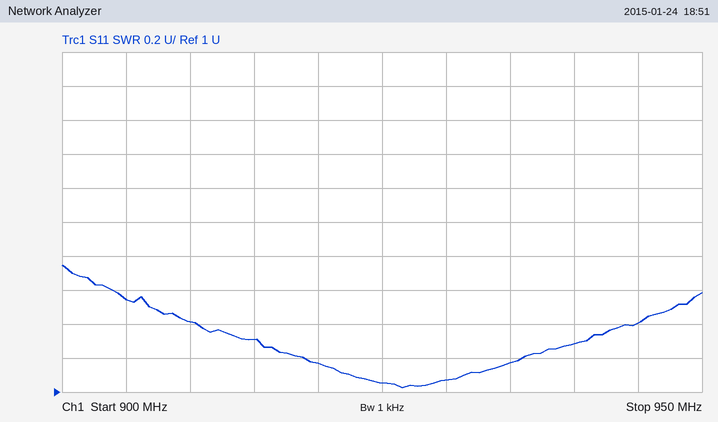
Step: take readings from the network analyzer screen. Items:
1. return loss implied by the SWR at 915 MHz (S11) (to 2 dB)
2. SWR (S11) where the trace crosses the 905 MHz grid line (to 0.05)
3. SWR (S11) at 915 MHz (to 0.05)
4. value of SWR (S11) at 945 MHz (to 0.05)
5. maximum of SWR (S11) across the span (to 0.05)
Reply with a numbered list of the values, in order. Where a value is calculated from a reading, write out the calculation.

1. −20 log10((1.3 − 1)/(1.3 + 1)) ≈ 18 dB
2. 1.55
3. 1.30
4. 1.40
5. 1.75
